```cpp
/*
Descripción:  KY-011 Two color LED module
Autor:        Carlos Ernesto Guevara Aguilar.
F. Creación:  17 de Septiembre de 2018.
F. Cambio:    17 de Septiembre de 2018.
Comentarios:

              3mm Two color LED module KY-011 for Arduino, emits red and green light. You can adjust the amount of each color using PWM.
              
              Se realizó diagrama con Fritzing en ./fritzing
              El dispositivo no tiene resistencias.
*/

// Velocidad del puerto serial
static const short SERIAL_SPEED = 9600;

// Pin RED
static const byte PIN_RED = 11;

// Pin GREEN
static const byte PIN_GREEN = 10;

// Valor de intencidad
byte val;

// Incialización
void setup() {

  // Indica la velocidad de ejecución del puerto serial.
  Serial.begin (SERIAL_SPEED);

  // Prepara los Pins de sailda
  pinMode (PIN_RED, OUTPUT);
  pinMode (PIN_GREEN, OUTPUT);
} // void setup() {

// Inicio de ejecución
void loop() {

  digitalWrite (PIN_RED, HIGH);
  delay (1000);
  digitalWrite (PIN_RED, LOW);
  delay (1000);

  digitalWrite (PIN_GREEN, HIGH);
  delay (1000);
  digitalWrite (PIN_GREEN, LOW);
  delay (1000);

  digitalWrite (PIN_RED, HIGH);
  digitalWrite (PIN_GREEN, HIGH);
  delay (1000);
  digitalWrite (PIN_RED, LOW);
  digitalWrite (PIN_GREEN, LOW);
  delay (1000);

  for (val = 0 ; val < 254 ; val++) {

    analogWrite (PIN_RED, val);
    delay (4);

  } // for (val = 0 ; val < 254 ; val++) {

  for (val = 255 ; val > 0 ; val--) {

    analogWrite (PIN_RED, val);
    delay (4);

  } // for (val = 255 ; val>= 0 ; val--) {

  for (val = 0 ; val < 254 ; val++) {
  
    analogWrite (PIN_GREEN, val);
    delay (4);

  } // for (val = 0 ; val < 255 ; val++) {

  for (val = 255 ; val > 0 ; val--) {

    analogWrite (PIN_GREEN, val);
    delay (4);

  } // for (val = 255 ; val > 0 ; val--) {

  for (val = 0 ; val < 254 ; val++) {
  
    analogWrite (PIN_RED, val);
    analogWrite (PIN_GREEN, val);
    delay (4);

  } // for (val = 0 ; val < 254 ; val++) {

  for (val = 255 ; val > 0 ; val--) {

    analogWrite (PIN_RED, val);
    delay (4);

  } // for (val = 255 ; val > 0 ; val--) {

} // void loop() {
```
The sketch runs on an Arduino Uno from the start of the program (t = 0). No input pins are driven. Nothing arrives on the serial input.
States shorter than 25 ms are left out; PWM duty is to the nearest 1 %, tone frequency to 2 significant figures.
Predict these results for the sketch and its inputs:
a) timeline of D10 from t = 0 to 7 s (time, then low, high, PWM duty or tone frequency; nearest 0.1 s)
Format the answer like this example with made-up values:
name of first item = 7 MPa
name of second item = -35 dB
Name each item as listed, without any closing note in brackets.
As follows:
timeline of D10 from t = 0 to 7 s = 0 s low; 2 s high; 3 s low; 4 s high; 5 s low
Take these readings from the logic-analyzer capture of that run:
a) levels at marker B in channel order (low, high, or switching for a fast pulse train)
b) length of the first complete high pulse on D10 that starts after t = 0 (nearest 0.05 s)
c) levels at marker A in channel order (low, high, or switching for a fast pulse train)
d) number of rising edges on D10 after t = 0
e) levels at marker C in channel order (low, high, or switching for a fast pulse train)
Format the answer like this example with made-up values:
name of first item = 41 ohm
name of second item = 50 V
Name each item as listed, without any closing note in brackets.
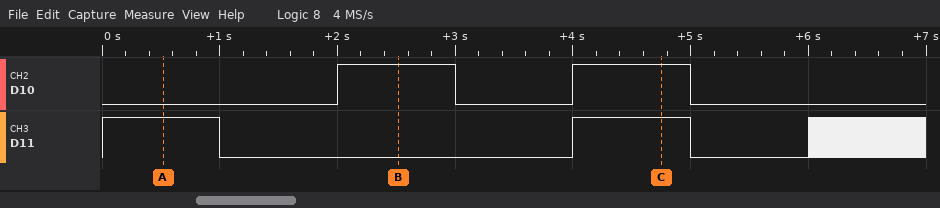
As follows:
levels at marker B in channel order = D10 high, D11 low
length of the first complete high pulse on D10 that starts after t = 0 = 1.00 s
levels at marker A in channel order = D10 low, D11 high
number of rising edges on D10 after t = 0 = 2
levels at marker C in channel order = D10 high, D11 high
